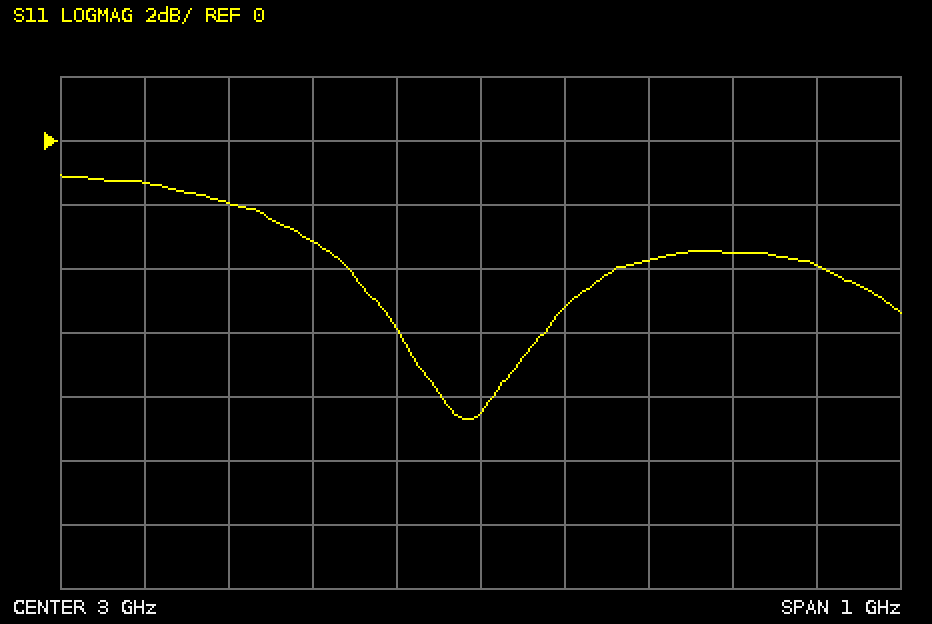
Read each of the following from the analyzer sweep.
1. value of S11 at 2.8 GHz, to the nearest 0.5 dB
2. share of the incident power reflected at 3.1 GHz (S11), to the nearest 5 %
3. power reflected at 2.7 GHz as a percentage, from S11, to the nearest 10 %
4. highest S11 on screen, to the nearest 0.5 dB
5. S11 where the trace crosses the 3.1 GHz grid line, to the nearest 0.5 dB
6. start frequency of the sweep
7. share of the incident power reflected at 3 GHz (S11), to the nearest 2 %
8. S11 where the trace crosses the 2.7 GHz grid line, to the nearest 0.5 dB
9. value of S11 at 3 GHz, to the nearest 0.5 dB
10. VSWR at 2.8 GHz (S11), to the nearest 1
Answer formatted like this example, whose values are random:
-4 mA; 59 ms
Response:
-3.0 dB; 30 %; 60 %; -1.0 dB; -5.0 dB; 2.5 GHz; 14 %; -2.0 dB; -8.5 dB; 6
